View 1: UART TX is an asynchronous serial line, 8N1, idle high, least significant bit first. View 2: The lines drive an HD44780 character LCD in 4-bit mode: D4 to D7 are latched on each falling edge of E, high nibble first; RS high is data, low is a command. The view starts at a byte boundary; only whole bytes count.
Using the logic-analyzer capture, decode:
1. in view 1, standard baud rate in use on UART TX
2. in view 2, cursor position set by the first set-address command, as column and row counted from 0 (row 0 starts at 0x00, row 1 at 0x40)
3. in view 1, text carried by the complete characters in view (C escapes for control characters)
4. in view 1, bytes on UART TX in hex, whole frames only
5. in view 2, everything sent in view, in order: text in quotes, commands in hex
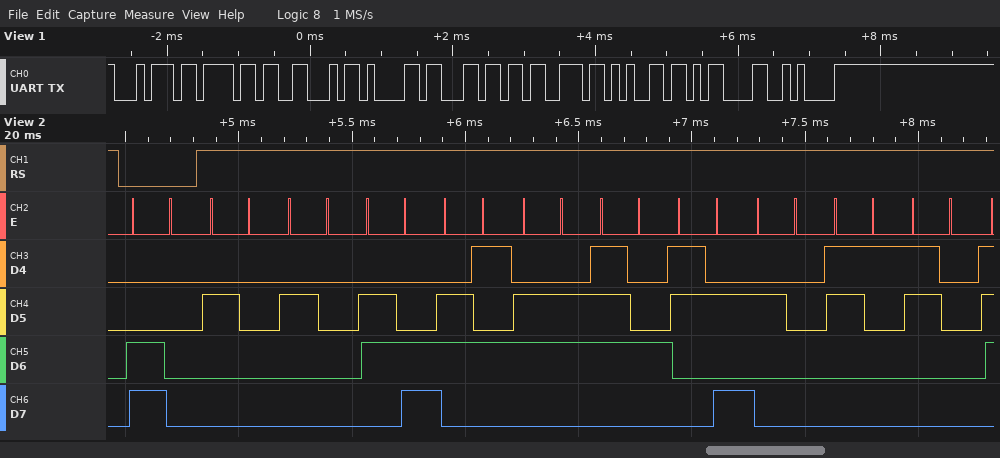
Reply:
9600 baud
column 0, row 1
"toFalse\r\n"
74 6F 46 61 6C 73 65 0D 0A
0xC0 "  left: 10"
